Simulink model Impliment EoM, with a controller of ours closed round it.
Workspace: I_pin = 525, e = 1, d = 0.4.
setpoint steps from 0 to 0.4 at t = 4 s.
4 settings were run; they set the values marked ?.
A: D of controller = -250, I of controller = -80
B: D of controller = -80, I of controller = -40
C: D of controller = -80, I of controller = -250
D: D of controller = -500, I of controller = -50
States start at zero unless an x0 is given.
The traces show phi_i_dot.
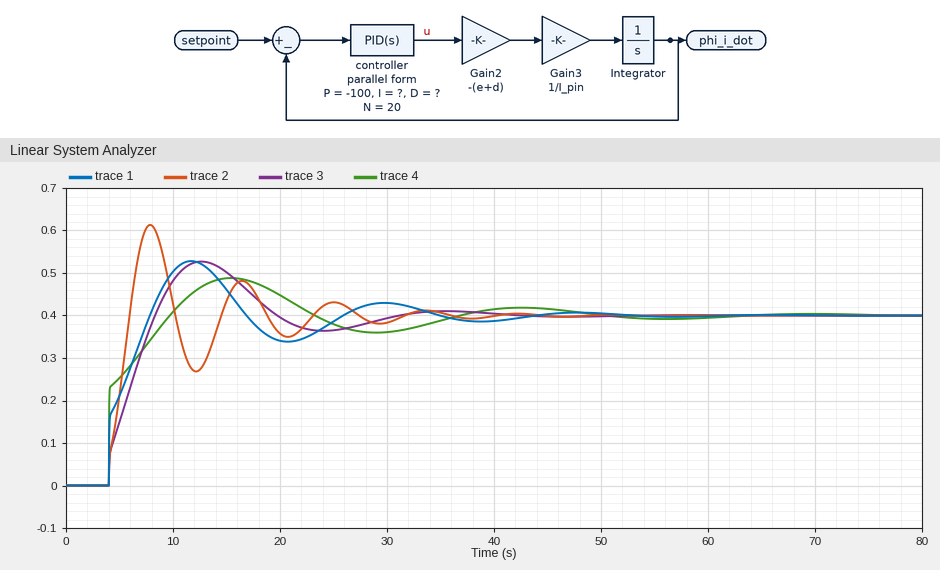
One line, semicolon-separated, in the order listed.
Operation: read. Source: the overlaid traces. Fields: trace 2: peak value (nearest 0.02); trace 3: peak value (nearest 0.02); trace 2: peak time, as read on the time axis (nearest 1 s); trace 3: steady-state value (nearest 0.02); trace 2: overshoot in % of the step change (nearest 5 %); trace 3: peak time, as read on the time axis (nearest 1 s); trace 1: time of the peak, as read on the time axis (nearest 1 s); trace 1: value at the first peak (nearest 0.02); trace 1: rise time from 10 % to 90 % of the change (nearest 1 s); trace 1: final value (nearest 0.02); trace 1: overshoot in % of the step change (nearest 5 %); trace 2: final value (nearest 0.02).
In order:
0.62; 0.52; 8 s; 0.40; 55 %; 13 s; 12 s; 0.52; 3 s; 0.40; 30 %; 0.40
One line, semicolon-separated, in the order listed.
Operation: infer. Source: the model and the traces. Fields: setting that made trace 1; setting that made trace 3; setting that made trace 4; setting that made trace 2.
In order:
A; B; D; C
